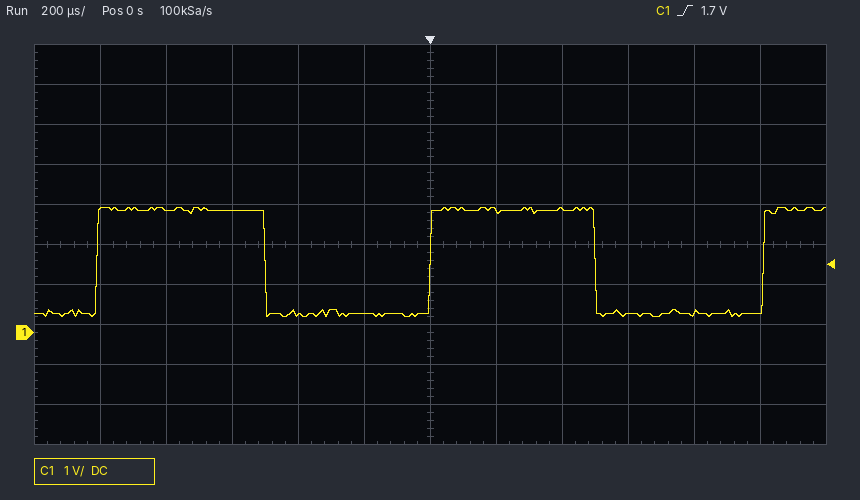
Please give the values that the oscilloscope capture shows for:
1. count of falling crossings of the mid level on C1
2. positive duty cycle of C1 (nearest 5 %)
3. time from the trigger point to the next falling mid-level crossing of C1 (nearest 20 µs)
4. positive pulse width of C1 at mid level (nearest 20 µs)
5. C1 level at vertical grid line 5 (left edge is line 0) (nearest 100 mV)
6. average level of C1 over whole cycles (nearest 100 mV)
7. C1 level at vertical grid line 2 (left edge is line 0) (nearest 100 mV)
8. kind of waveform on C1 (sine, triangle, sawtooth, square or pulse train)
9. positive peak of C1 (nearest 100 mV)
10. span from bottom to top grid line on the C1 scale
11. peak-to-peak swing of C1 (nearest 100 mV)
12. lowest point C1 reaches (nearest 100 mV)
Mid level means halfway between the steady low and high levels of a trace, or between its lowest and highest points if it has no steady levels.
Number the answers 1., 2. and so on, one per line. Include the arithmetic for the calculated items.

1. 2
2. 50 %
3. 500 µs
4. 500 µs
5. 500 mV
6. 400 mV + 0.5 × (3.1 V − (400 mV)) ≈ 1.8 V
7. 3.1 V
8. square
9. 3.1 V
10. 10 V
11. 3.1 V − (400 mV) = 2.7 V
12. 400 mV
